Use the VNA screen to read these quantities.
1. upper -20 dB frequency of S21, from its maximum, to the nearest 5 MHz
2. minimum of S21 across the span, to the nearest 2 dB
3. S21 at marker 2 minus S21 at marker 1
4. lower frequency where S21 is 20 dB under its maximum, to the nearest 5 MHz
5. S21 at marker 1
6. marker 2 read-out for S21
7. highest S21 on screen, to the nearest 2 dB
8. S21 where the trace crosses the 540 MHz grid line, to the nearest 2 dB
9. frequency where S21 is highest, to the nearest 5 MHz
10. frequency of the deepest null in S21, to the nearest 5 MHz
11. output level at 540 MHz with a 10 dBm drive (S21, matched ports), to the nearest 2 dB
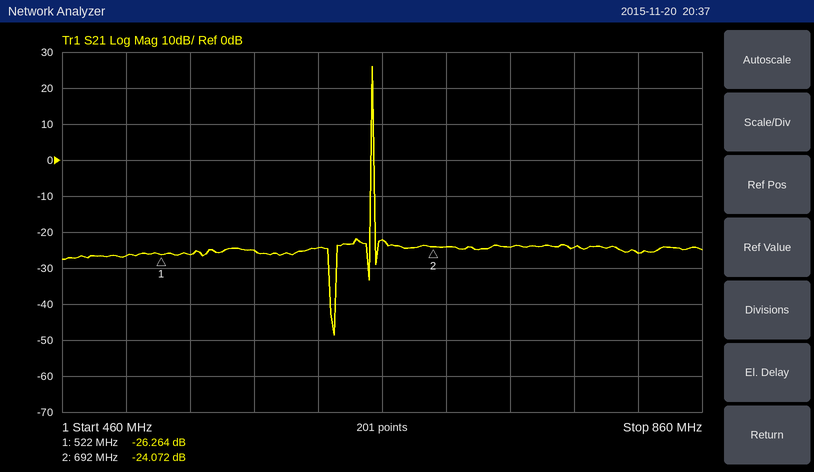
655 MHz
-48 dB
2.192 dB
655 MHz
-26.264 dB
-24.072 dB
26 dB
-26 dB
655 MHz
630 MHz
-16 dBm
